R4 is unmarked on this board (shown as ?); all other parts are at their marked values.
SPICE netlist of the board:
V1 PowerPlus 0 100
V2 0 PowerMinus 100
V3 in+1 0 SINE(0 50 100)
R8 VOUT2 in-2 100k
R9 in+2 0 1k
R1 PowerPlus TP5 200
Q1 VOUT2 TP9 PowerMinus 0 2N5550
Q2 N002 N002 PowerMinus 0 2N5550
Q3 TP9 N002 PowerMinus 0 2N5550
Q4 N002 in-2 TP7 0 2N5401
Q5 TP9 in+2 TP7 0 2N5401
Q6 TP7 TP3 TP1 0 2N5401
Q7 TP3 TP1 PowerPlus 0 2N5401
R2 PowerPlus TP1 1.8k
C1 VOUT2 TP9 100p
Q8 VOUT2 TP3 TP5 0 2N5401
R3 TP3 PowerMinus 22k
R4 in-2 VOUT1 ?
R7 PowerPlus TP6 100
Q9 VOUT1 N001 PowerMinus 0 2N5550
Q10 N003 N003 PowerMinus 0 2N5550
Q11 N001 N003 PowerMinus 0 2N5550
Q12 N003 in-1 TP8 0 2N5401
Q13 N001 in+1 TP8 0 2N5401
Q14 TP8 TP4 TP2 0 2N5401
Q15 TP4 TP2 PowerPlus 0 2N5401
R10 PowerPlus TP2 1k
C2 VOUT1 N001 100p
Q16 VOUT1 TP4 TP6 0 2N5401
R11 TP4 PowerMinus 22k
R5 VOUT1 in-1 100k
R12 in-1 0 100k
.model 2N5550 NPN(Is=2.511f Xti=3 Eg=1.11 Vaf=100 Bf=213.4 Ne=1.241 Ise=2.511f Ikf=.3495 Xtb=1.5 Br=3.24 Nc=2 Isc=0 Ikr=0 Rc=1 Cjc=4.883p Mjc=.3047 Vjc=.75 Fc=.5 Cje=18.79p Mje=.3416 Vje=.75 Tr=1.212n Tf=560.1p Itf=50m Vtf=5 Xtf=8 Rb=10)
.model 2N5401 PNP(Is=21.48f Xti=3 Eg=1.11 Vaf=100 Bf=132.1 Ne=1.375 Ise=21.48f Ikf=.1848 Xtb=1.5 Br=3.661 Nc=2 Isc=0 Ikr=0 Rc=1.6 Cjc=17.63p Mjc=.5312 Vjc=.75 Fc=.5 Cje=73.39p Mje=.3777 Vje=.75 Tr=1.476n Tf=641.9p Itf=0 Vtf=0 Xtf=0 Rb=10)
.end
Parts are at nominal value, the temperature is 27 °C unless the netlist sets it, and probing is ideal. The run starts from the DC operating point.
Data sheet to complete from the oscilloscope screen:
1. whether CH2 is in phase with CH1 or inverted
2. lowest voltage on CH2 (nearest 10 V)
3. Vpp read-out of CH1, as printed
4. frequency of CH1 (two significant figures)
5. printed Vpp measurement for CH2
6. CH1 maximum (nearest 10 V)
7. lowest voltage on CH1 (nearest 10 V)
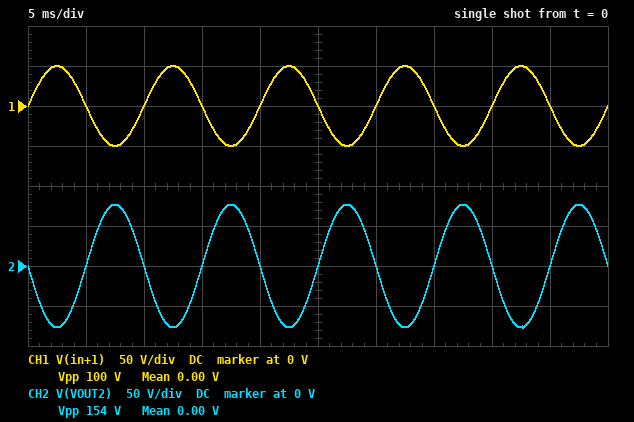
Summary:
inverted
-80 V
100 V
100 Hz
154 V
50 V
-50 V
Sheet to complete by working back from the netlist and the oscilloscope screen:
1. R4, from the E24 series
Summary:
130 kΩ
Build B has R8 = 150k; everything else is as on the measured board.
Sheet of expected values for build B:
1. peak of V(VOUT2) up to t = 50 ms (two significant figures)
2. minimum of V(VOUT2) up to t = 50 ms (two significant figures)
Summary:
99 V
-100 V
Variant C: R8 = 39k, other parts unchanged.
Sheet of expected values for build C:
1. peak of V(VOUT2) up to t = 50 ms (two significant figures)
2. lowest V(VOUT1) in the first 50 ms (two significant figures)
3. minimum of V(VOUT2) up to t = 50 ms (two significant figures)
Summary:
30 V
-100 V
-30 V
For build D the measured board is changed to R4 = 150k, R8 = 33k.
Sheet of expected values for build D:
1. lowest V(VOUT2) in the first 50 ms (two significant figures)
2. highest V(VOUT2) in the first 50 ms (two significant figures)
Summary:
-22 V
22 V
